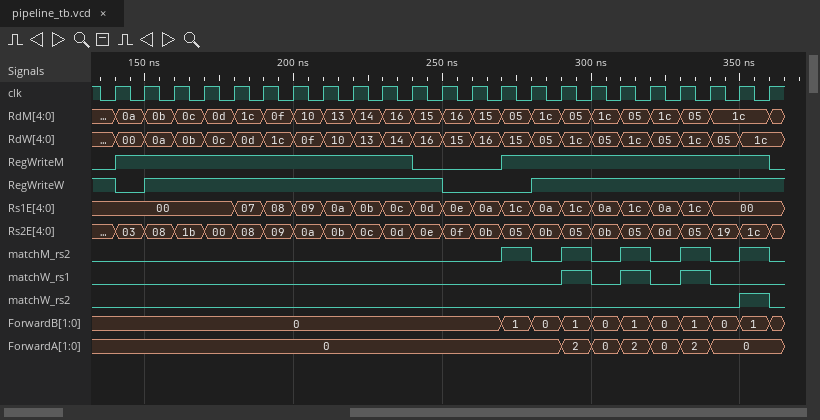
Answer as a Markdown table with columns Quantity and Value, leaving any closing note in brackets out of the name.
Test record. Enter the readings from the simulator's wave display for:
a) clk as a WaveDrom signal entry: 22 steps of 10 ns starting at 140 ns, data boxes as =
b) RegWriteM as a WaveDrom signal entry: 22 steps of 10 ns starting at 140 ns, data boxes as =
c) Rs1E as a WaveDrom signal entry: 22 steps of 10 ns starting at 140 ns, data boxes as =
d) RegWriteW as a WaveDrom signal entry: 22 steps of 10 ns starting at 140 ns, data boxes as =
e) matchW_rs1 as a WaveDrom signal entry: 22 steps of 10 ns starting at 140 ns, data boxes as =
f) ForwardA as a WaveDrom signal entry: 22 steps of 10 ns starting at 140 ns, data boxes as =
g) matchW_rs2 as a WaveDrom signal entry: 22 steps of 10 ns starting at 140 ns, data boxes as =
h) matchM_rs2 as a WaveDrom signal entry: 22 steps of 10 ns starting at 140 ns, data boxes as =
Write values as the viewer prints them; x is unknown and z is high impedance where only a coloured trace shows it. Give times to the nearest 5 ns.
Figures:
| Quantity | Value |
|---|---|
| clk as a WaveDrom signal entry: 22 steps of 10 ns starting at 140 ns, data boxes as = | {name: 'clk', wave: 'p.....................'} |
| RegWriteM as a WaveDrom signal entry: 22 steps of 10 ns starting at 140 ns, data boxes as = | {name: 'RegWriteM', wave: '1.........0..1........'} |
| Rs1E as a WaveDrom signal entry: 22 steps of 10 ns starting at 140 ns, data boxes as = | {name: 'Rs1E', wave: '=...=================.', data: '00 07 08 09 0a 0b 0c 0d 0e 0a 1c 0a 1c 0a 1c 0a 1c 00'} |
| RegWriteW as a WaveDrom signal entry: 22 steps of 10 ns starting at 140 ns, data boxes as = | {name: 'RegWriteW', wave: '01.........0..1.......'} |
| matchW_rs1 as a WaveDrom signal entry: 22 steps of 10 ns starting at 140 ns, data boxes as = | {name: 'matchW_rs1', wave: '0..............101010.'} |
| ForwardA as a WaveDrom signal entry: 22 steps of 10 ns starting at 140 ns, data boxes as = | {name: 'ForwardA', wave: '=..............======.', data: '0 2 0 2 0 2 0'} |
| matchW_rs2 as a WaveDrom signal entry: 22 steps of 10 ns starting at 140 ns, data boxes as = | {name: 'matchW_rs2', wave: '0....................1'} |
| matchM_rs2 as a WaveDrom signal entry: 22 steps of 10 ns starting at 140 ns, data boxes as = | {name: 'matchM_rs2', wave: '0............101010101'} |
